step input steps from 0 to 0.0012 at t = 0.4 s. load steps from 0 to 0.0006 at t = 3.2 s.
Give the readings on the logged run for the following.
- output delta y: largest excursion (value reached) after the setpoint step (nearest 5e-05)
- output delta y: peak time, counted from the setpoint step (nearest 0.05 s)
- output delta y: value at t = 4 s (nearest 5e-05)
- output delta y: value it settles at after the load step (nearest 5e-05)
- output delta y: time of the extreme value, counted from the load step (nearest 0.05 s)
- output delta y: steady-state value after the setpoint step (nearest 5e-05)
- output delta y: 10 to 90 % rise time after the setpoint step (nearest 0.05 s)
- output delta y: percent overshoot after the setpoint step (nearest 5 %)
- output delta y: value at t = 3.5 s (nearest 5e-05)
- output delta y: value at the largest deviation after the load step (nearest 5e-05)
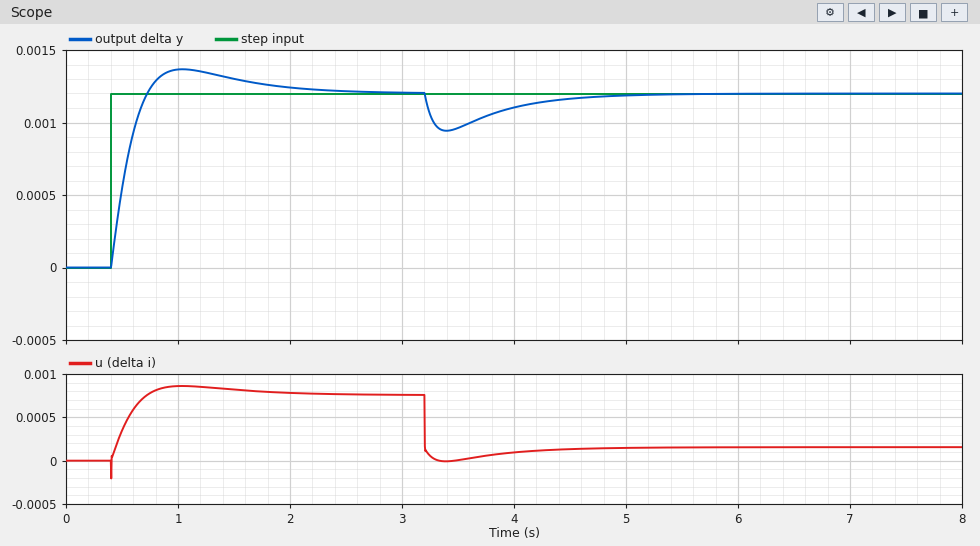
0.00135
0.65 s
0.00110
0.00120
0.20 s
0.00120
0.25 s
15 %
0.00095
0.00095
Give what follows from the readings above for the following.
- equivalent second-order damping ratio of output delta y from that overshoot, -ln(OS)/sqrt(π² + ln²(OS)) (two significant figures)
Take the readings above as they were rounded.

0.52
